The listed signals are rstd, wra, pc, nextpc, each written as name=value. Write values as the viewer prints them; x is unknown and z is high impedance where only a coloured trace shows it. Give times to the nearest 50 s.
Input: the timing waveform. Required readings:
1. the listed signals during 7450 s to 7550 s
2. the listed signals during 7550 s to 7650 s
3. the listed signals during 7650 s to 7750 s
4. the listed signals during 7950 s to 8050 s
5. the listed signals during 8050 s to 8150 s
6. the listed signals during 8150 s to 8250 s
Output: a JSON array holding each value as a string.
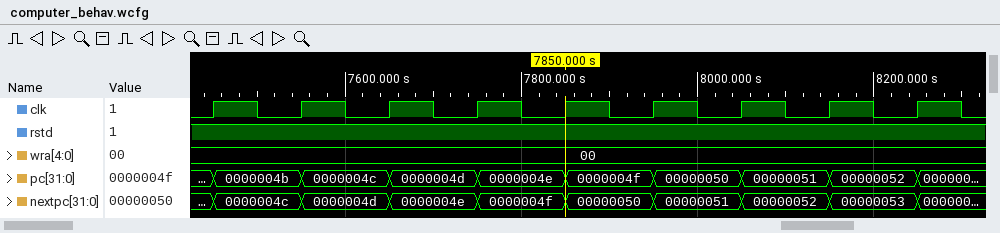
["rstd=1, wra=00, pc=0000004b, nextpc=0000004c", "rstd=1, wra=00, pc=0000004c, nextpc=0000004d", "rstd=1, wra=00, pc=0000004d, nextpc=0000004e", "rstd=1, wra=00, pc=00000050, nextpc=00000051", "rstd=1, wra=00, pc=00000051, nextpc=00000052", "rstd=1, wra=00, pc=00000052, nextpc=00000053"]
